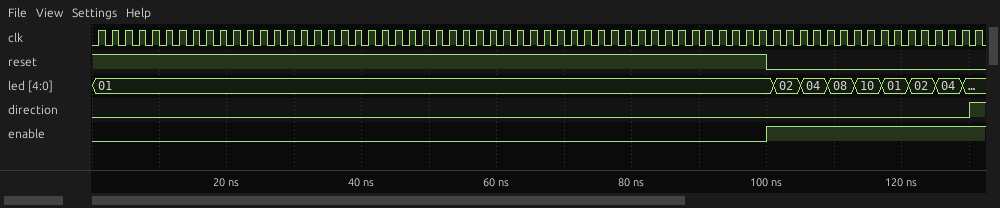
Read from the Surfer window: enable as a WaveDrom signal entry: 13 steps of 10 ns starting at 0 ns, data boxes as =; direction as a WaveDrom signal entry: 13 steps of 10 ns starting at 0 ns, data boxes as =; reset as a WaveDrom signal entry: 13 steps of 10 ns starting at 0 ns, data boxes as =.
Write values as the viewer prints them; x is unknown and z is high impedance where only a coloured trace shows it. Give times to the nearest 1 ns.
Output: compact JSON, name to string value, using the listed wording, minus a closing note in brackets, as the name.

{"enable as a WaveDrom signal entry: 13 steps of 10 ns starting at 0 ns, data boxes as =": "{name: 'enable', wave: '0.........1..'}", "direction as a WaveDrom signal entry: 13 steps of 10 ns starting at 0 ns, data boxes as =": "{name: 'direction', wave: '0............'}", "reset as a WaveDrom signal entry: 13 steps of 10 ns starting at 0 ns, data boxes as =": "{name: 'reset', wave: '1.........0..'}"}
